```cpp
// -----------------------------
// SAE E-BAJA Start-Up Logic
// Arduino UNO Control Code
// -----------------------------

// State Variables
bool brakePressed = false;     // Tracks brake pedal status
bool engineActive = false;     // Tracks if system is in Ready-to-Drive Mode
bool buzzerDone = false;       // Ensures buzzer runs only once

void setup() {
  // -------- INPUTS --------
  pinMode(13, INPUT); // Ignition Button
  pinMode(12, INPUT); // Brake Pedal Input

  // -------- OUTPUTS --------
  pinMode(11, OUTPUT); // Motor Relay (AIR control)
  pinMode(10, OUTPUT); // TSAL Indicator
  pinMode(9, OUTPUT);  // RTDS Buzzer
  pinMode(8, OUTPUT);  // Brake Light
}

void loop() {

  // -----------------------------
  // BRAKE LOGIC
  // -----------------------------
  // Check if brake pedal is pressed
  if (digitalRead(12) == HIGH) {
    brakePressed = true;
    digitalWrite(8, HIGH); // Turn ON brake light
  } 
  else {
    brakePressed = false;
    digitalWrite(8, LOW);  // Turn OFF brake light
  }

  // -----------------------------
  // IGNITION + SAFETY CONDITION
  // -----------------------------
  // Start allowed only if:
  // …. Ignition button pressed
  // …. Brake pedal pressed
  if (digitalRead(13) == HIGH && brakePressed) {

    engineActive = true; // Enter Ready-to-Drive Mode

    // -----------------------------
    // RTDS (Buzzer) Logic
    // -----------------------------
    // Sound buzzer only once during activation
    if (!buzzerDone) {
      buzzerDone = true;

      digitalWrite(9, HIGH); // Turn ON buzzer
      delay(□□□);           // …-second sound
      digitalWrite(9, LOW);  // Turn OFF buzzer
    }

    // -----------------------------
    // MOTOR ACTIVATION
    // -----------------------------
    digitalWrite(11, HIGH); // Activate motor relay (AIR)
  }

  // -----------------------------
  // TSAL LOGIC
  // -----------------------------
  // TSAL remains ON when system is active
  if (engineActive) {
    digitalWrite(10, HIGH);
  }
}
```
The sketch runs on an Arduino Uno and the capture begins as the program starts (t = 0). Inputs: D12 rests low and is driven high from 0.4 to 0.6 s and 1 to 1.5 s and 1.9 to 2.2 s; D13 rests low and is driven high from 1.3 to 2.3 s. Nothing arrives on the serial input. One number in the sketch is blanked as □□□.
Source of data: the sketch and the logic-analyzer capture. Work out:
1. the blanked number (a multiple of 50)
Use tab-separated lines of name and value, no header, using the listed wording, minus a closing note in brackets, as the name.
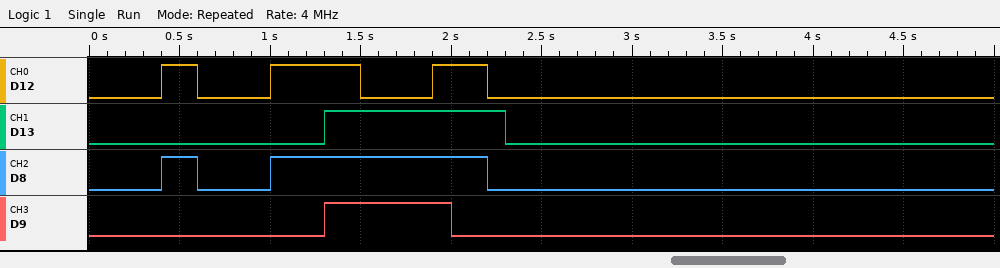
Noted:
the blanked number	700
